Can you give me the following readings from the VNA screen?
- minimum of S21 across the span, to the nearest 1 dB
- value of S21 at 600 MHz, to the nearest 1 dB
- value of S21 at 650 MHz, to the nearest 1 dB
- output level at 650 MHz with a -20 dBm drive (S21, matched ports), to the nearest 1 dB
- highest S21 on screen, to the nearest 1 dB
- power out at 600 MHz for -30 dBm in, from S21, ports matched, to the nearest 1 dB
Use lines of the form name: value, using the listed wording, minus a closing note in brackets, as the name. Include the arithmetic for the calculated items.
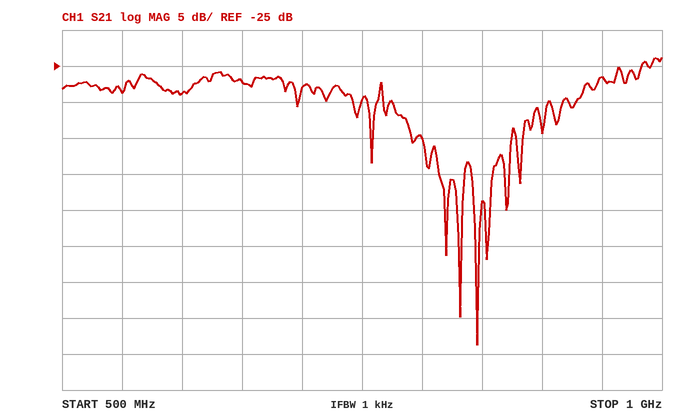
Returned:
minimum of S21 across the span, to the nearest 1 dB: -64 dB
value of S21 at 600 MHz, to the nearest 1 dB: -29 dB
value of S21 at 650 MHz, to the nearest 1 dB: -27 dB
output level at 650 MHz with a -20 dBm drive (S21, matched ports), to the nearest 1 dB: -20 dBm + (-27 dB) = -47 dBm
highest S21 on screen, to the nearest 1 dB: -24 dB
power out at 600 MHz for -30 dBm in, from S21, ports matched, to the nearest 1 dB: -30 dBm + (-29 dB) = -59 dBm
